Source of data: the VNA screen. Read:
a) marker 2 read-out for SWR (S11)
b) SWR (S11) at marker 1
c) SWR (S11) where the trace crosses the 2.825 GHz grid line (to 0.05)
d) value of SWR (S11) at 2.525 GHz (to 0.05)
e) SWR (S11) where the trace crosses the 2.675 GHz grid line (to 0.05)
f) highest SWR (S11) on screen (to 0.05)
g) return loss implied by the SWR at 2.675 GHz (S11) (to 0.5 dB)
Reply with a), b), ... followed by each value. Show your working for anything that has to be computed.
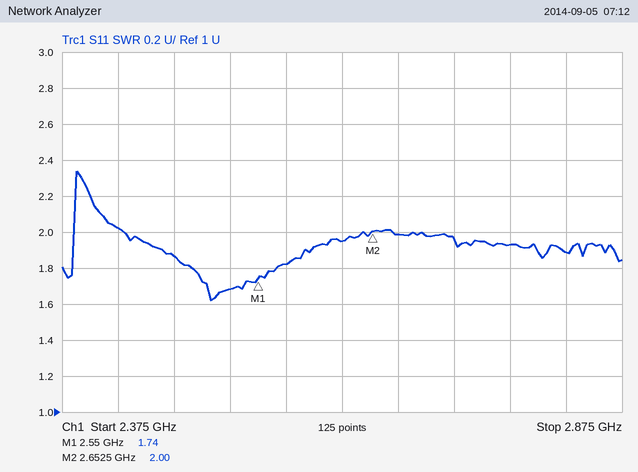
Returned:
a) 2.00
b) 1.74
c) 1.90
d) 1.70
e) 2.00
f) 2.35
g) −20 log10((2 − 1)/(2 + 1)) ≈ 9.5 dB
